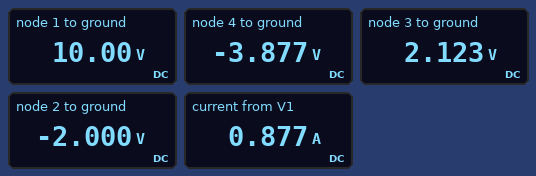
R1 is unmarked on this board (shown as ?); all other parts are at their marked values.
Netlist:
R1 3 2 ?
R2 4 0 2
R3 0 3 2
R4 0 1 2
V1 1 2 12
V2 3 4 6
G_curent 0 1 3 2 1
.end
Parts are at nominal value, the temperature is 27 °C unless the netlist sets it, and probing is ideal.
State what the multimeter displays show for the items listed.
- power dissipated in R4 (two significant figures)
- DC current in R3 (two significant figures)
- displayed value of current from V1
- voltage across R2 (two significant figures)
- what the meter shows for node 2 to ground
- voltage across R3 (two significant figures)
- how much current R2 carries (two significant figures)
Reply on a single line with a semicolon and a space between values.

50 W; 1.1 A; 0.877 A; 3.9 V; -2.000 V; 2.1 V; 1.9 A
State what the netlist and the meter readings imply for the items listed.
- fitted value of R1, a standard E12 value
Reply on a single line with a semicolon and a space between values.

4.7 Ω
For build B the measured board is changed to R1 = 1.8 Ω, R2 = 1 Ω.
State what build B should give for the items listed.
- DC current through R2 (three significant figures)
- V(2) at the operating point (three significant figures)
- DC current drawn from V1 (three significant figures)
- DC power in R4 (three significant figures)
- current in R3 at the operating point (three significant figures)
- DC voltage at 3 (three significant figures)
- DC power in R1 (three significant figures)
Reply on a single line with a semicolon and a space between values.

3.32 A; -893 mV; 1.98 A; 61.7 W; 1.34 A; 2.68 V; 7.08 W
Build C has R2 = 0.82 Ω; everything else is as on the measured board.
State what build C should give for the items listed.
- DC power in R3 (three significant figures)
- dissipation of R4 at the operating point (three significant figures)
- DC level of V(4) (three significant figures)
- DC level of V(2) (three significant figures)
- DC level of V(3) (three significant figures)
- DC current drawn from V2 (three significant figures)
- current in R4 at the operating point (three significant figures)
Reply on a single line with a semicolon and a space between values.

6.80 W; 61.7 W; -2.31 V; -891 mV; 3.69 V; 2.82 A; 5.55 A
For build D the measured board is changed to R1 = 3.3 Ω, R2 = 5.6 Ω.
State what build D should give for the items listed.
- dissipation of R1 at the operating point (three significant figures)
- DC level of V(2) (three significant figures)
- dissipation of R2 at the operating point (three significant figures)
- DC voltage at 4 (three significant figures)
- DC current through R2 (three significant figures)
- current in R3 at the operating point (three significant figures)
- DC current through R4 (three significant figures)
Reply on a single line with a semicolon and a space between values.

3.40 W; -3.27 V; 6.25 W; -5.92 V; 1.06 A; 41.3 mA; 4.37 A
